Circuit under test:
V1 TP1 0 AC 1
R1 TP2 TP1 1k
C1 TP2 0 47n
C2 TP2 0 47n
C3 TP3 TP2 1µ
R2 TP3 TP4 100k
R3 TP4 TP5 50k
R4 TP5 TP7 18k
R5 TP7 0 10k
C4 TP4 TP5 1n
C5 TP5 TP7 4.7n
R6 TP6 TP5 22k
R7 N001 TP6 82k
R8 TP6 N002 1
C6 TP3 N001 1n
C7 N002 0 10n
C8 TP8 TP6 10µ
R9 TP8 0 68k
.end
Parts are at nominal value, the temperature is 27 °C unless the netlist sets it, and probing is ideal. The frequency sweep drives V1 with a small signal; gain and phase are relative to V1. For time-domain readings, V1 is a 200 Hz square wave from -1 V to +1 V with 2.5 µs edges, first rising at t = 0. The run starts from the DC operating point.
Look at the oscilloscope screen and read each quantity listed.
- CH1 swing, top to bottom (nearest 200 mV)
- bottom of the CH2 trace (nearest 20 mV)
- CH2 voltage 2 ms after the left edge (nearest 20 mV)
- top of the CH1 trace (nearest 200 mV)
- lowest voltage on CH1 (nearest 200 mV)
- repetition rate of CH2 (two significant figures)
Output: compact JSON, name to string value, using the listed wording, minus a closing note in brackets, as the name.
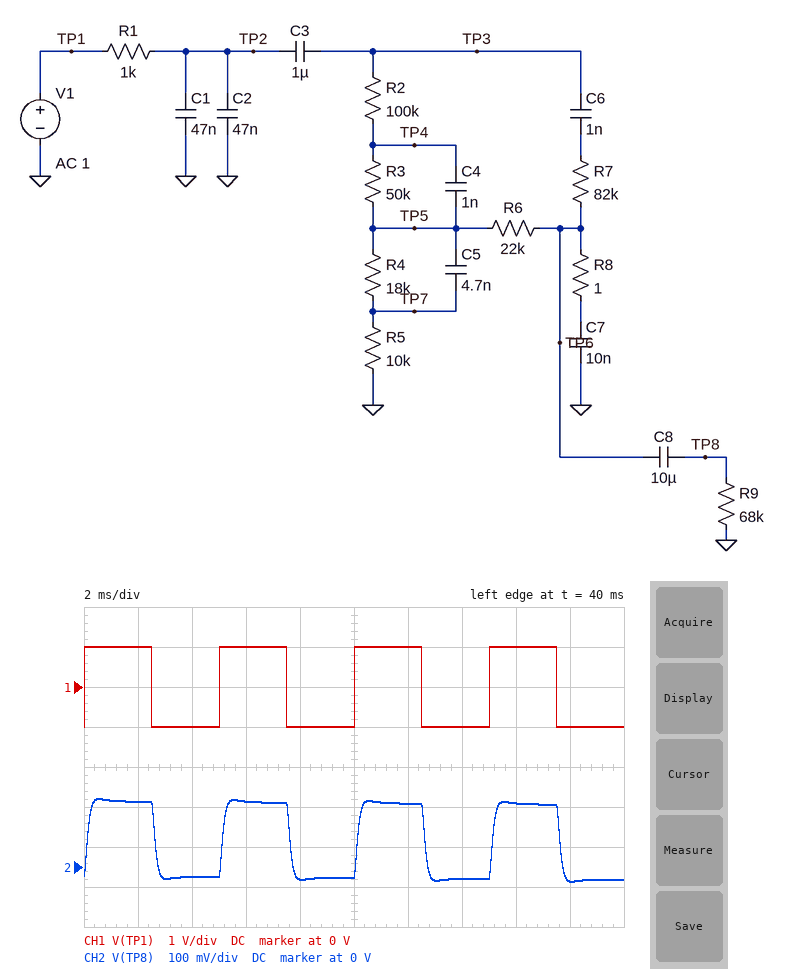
{"CH1 swing, top to bottom": "2.0 V", "bottom of the CH2 trace": "-40 mV", "CH2 voltage 2 ms after the left edge": "160 mV", "top of the CH1 trace": "1.0 V", "lowest voltage on CH1": "-1.0 V", "repetition rate of CH2": "200 Hz"}
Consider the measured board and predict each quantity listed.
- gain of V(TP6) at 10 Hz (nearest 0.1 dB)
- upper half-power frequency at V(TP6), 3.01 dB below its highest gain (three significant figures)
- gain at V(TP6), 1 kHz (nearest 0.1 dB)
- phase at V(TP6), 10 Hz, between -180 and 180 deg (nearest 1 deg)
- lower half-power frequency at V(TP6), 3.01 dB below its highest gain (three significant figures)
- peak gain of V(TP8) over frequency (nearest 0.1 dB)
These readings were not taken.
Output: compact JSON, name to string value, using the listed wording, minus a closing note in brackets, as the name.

{"gain of V(TP6) at 10 Hz": "-20.6 dB", "upper half-power frequency at V(TP6), 3.01 dB below its highest gain": "1.42 kHz", "gain at V(TP6), 1 kHz": "-21.9 dB", "phase at V(TP6), 10 Hz, between -180 and 180 deg": "4 deg", "lower half-power frequency at V(TP6), 3.01 dB below its highest gain": "905 mHz", "peak gain of V(TP8) over frequency": "-20.5 dB"}
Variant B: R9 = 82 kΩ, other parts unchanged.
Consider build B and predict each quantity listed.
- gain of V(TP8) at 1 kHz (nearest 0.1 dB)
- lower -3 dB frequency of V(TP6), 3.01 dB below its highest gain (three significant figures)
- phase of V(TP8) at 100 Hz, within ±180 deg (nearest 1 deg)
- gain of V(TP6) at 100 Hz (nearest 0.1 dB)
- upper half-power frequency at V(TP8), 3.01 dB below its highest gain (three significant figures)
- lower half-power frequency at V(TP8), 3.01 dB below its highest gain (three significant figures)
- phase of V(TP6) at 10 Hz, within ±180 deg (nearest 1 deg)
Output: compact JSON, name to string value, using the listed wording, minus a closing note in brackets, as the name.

{"gain of V(TP8) at 1 kHz": "-21.8 dB", "lower -3 dB frequency of V(TP6), 3.01 dB below its highest gain": "898 mHz", "phase of V(TP8) at 100 Hz, within ±180 deg": "-5 deg", "gain of V(TP6) at 100 Hz": "-20.0 dB", "upper half-power frequency at V(TP8), 3.01 dB below its highest gain": "1.31 kHz", "lower half-power frequency at V(TP8), 3.01 dB below its highest gain": "938 mHz", "phase of V(TP6) at 10 Hz, within ±180 deg": "4 deg"}
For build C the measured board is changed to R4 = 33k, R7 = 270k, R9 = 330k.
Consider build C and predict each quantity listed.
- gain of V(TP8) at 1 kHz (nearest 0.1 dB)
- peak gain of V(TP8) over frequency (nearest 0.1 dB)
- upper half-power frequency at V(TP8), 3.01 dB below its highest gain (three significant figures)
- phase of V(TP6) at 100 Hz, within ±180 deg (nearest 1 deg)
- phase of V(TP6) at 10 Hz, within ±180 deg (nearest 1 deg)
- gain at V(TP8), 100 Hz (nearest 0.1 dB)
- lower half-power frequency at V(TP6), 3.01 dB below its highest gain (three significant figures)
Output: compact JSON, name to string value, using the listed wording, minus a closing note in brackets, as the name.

{"gain of V(TP8) at 1 kHz": "-22.4 dB", "peak gain of V(TP8) over frequency": "-14.5 dB", "upper half-power frequency at V(TP8), 3.01 dB below its highest gain": "442 Hz", "phase of V(TP6) at 100 Hz, within ±180 deg": "-15 deg", "phase of V(TP6) at 10 Hz, within ±180 deg": "3 deg", "gain at V(TP8), 100 Hz": "-14.7 dB", "lower half-power frequency at V(TP6), 3.01 dB below its highest gain": "836 mHz"}
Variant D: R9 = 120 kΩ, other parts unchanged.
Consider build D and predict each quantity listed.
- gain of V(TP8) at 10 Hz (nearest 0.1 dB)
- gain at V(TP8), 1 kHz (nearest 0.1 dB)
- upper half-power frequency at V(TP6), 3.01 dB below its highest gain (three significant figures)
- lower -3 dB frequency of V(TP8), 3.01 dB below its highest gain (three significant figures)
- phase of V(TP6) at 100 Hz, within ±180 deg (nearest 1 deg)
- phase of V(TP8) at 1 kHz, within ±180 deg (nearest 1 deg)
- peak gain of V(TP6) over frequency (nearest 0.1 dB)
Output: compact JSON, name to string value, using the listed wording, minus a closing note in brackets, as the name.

{"gain of V(TP8) at 10 Hz": "-19.0 dB", "gain at V(TP8), 1 kHz": "-21.6 dB", "upper half-power frequency at V(TP6), 3.01 dB below its highest gain": "1.09 kHz", "lower -3 dB frequency of V(TP8), 3.01 dB below its highest gain": "922 mHz", "phase of V(TP6) at 100 Hz, within ±180 deg": "-6 deg", "phase of V(TP8) at 1 kHz, within ±180 deg": "-56 deg", "peak gain of V(TP6) over frequency": "-18.9 dB"}
